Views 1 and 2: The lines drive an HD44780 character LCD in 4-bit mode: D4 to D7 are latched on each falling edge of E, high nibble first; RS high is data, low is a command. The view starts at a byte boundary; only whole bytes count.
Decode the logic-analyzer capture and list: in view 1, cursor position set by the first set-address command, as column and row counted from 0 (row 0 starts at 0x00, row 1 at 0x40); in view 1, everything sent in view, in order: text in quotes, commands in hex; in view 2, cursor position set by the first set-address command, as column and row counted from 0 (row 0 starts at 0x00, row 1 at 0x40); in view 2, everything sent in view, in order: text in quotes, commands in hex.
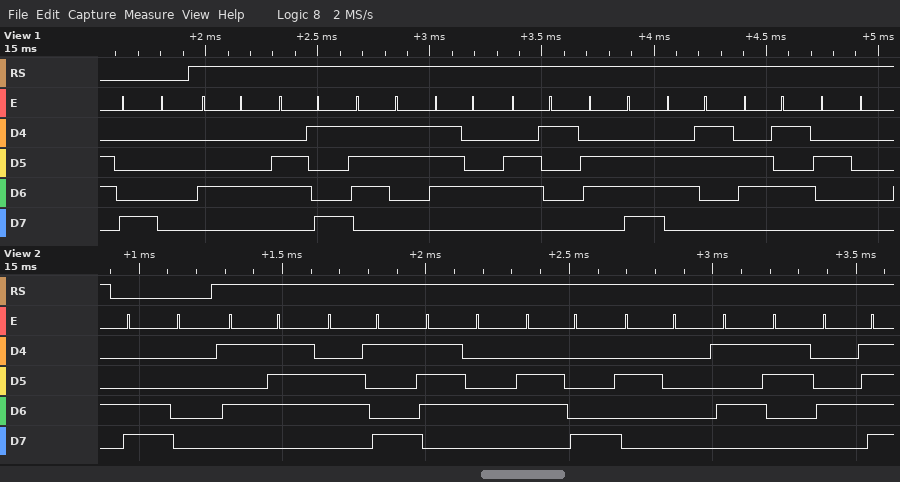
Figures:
column 0, row 0
0x80 "Distance "
column 0, row 1
0xC0 "With SO"
